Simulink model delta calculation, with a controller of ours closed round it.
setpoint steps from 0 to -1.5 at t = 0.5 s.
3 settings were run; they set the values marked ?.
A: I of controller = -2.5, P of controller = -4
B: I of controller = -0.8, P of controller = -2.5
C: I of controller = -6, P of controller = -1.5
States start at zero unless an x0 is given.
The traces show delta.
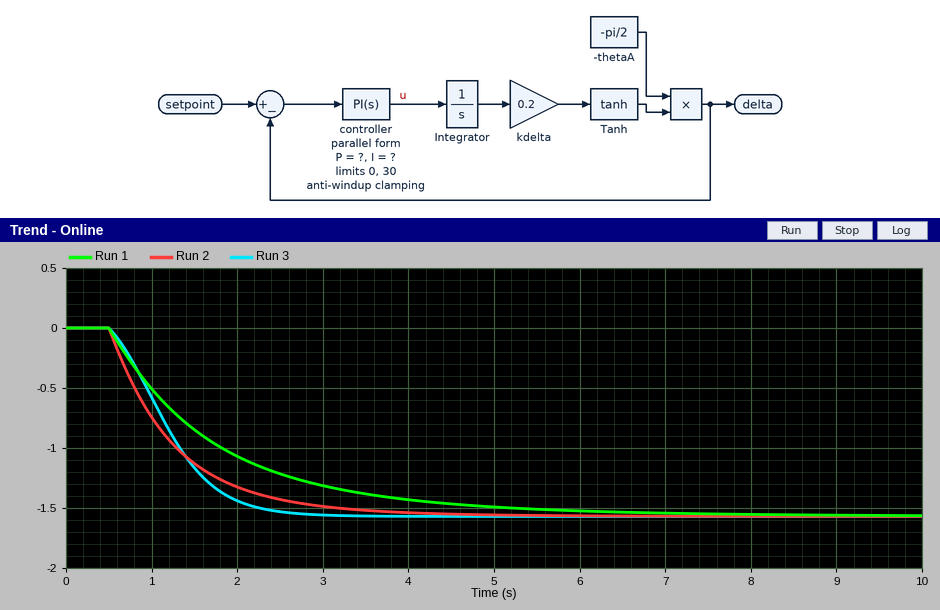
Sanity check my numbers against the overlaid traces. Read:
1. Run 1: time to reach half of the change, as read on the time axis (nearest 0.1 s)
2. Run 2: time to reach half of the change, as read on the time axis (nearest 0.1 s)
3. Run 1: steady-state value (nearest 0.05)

1.4 s
1.0 s
-1.55
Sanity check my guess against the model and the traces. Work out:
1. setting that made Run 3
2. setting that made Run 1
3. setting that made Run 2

C
B
A
